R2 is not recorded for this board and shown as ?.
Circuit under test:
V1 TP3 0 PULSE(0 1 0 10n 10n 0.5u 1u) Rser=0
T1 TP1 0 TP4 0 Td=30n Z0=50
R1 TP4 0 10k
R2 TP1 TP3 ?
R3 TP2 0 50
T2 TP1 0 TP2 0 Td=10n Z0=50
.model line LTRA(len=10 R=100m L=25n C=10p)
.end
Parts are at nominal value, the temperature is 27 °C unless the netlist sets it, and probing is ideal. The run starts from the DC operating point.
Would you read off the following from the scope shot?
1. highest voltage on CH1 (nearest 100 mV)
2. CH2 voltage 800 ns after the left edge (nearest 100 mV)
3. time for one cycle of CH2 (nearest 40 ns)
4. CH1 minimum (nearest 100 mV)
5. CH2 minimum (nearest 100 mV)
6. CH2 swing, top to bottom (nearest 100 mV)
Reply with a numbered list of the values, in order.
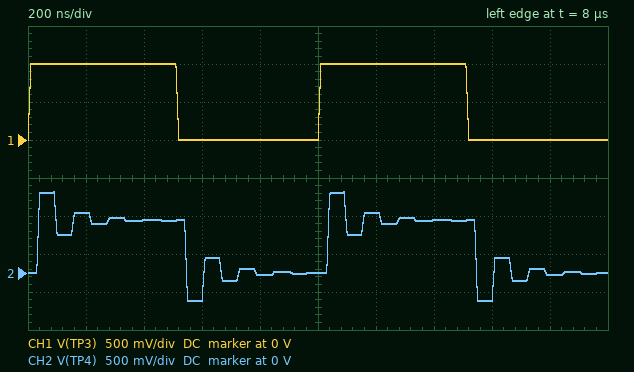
1. 1.0 V
2. 0 V
3. 1.00 µs
4. 0 V
5. -400 mV
6. 1.4 V
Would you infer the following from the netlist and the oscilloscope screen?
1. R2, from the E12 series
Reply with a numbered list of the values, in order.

1. 22 Ω
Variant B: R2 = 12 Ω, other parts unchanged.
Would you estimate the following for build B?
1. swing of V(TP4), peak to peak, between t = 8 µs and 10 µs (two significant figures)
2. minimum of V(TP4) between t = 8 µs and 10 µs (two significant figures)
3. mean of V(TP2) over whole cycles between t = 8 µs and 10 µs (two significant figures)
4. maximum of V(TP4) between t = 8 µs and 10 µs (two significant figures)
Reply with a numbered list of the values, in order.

1. 1.9 V
2. -550 mV
3. 410 mV
4. 1.4 V
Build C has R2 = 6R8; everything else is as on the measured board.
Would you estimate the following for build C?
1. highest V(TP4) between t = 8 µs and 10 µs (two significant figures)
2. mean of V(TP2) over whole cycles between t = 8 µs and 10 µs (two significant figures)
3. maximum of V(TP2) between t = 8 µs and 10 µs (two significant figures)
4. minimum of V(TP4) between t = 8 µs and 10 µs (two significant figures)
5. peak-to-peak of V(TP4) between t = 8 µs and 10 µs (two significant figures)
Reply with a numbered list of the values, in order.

1. 1.6 V
2. 450 mV
3. 960 mV
4. -750 mV
5. 2.4 V
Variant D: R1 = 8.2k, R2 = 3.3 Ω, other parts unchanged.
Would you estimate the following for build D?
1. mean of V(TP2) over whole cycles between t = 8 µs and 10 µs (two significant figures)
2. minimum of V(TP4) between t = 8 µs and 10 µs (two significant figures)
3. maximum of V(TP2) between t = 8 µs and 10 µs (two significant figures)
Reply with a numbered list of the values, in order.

1. 480 mV
2. -1.0 V
3. 1.0 V
